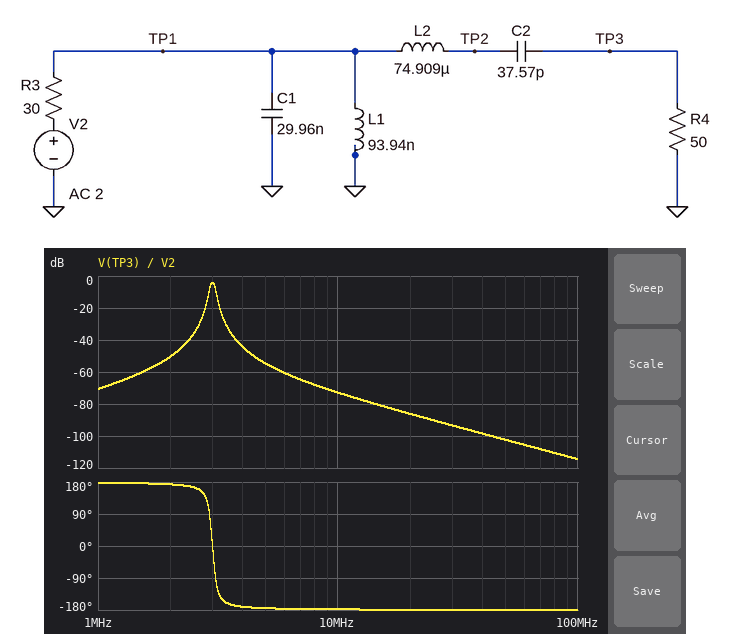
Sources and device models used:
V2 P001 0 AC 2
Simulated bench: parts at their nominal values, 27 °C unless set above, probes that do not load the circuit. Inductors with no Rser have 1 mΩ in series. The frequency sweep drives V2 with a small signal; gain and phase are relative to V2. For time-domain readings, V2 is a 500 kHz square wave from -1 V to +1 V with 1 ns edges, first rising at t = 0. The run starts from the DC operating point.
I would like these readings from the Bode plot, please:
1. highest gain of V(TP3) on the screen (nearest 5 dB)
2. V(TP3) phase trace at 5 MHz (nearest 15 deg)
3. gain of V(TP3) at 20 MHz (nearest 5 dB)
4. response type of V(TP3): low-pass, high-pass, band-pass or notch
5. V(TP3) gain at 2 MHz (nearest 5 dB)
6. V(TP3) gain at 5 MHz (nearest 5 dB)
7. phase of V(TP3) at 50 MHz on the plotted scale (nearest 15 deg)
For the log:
-5 dB
-180 deg
-85 dB
band-pass
-50 dB
-55 dB
-180 deg
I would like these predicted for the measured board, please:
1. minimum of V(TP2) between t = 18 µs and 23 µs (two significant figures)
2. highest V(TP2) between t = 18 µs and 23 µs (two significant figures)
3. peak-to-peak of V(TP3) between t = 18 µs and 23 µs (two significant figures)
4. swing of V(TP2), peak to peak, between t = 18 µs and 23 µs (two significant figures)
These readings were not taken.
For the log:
-270 mV
270 mV
17 mV
530 mV
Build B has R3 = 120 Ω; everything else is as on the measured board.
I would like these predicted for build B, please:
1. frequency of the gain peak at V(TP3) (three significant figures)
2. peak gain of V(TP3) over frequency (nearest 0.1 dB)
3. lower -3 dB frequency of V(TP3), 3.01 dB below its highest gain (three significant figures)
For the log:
2.97 MHz
-10.4 dB
2.93 MHz
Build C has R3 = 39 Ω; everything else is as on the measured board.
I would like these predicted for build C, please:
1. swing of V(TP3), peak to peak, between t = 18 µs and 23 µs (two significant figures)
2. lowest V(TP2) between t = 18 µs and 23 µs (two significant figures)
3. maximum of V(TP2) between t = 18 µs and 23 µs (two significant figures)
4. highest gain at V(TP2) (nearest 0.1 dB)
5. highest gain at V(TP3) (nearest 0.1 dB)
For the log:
13 mV
-210 mV
210 mV
24.0 dB
-5.1 dB
